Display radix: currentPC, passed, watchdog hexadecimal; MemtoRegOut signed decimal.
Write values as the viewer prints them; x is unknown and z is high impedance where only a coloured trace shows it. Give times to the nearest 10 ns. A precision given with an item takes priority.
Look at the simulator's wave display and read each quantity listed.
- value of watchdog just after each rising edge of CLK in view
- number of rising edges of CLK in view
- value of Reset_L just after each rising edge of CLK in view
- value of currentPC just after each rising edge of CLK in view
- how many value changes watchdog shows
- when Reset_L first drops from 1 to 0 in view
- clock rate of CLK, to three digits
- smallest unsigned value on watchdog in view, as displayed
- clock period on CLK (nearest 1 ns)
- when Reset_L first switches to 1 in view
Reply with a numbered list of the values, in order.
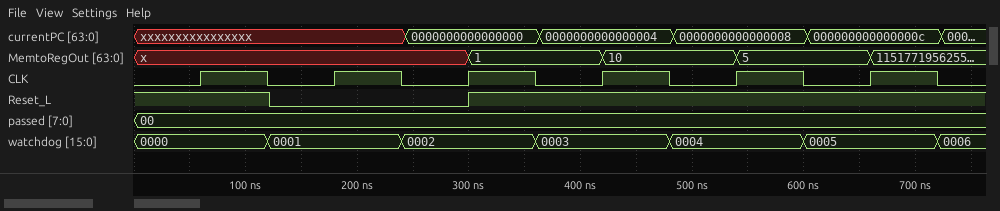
1. 0000, 0001, 0002, 0003, 0004, 0005
2. 6
3. 1 0 1 1 1 1
4. xxxxxxxxxxxxxxxx, xxxxxxxxxxxxxxxx, 0000000000000000, 0000000000000004, 0000000000000008, 000000000000000c
5. 6
6. 120 ns
7. 8.33 MHz
8. 0000
9. 120 ns
10. 300 ns
